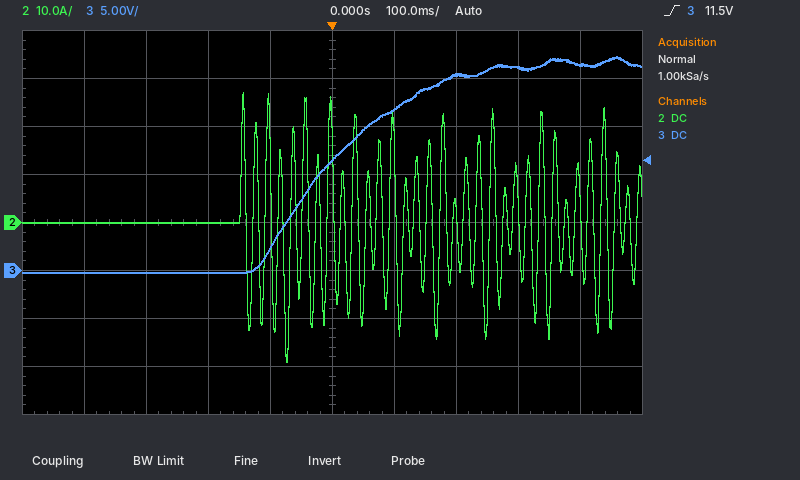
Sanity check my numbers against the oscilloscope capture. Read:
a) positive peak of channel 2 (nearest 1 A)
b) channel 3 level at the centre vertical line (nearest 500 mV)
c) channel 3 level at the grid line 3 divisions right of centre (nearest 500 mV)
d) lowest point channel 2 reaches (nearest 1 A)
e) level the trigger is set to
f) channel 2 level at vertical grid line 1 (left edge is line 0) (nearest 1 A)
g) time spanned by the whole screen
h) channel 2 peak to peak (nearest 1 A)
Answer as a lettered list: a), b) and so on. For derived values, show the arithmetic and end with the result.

a) 27 A
b) 11.5 V
c) 21.0 V
d) -29 A
e) 11.5 V
f) 0 A
g) 1 s
h) 27 A − (-29 A) = 56 A
